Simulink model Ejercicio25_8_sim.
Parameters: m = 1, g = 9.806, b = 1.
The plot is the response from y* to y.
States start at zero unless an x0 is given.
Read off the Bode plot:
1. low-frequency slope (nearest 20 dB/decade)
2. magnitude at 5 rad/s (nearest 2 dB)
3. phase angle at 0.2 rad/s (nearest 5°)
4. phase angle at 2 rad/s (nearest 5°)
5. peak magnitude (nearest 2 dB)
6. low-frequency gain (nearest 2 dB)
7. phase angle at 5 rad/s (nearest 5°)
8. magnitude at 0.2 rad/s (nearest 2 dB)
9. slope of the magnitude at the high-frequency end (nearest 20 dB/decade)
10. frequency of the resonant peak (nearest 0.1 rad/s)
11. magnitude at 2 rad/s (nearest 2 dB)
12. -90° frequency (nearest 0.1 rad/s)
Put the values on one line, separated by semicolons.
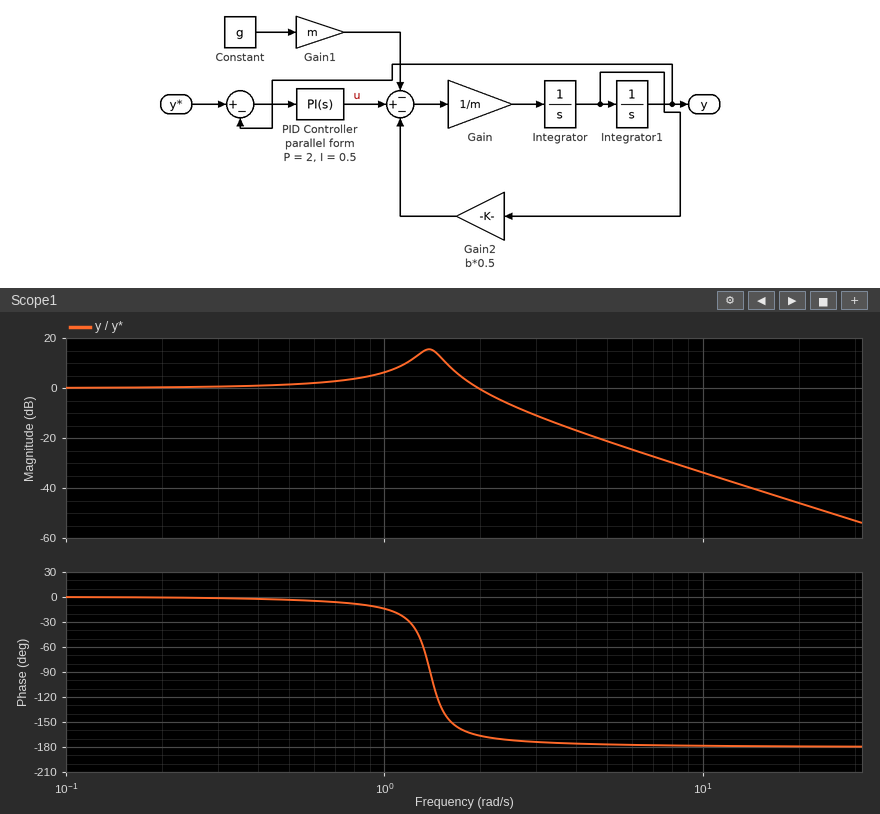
0 dB/decade; -22 dB; 0°; -165°; 16 dB; 0 dB; -175°; 0 dB; -40 dB/decade; 1.4 rad/s; 0 dB; 1.4 rad/s
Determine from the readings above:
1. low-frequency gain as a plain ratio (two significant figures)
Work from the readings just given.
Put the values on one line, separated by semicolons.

1.0
